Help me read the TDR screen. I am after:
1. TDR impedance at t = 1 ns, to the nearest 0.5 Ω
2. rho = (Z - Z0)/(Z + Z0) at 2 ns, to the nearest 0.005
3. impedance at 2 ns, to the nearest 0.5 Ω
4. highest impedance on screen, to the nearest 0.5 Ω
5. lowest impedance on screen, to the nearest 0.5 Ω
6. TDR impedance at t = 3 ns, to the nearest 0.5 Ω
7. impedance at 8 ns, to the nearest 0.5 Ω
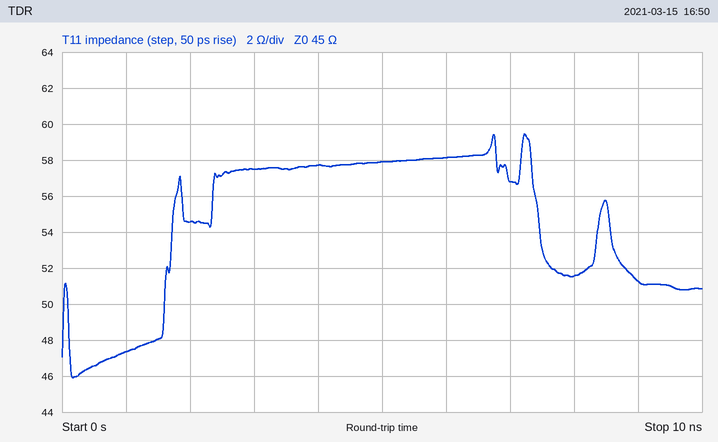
47.5 Ω
+0.095
54.5 Ω
59.5 Ω
46.0 Ω
57.5 Ω
51.5 Ω
